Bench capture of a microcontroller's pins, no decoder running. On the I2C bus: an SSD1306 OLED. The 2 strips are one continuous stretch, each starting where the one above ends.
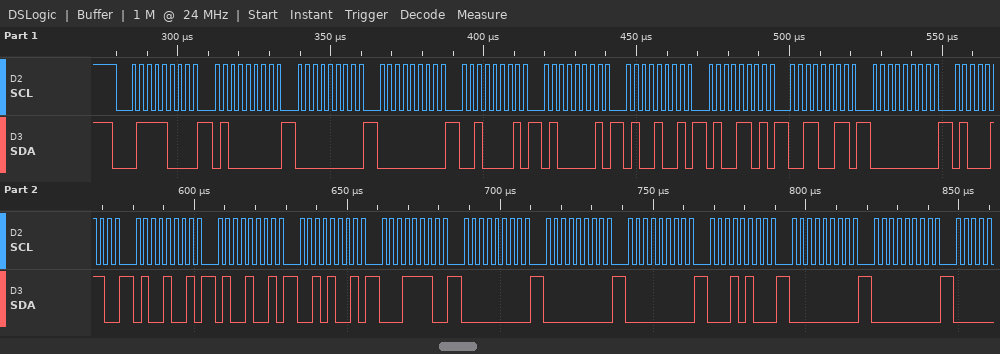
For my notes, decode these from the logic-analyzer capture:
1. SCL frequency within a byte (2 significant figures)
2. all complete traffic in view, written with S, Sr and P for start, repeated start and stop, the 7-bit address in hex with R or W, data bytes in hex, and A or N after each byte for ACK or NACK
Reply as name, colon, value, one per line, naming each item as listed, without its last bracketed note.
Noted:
SCL frequency within a byte: 400 kHz
all complete traffic in view, written with S, Sr and P for start, repeated start and stop, the 7-bit address in hex with R or W, data bytes in hex, and A or N after each byte for ACK or NACK: S 3CW A 40 A 00 A 00 A 21 A 41 A 49 A 4D A 33 A 00 A 46 A 49 A 49 A 29 A 1E A 00 A 00 A 00 A 14 A 00 A 00 A
